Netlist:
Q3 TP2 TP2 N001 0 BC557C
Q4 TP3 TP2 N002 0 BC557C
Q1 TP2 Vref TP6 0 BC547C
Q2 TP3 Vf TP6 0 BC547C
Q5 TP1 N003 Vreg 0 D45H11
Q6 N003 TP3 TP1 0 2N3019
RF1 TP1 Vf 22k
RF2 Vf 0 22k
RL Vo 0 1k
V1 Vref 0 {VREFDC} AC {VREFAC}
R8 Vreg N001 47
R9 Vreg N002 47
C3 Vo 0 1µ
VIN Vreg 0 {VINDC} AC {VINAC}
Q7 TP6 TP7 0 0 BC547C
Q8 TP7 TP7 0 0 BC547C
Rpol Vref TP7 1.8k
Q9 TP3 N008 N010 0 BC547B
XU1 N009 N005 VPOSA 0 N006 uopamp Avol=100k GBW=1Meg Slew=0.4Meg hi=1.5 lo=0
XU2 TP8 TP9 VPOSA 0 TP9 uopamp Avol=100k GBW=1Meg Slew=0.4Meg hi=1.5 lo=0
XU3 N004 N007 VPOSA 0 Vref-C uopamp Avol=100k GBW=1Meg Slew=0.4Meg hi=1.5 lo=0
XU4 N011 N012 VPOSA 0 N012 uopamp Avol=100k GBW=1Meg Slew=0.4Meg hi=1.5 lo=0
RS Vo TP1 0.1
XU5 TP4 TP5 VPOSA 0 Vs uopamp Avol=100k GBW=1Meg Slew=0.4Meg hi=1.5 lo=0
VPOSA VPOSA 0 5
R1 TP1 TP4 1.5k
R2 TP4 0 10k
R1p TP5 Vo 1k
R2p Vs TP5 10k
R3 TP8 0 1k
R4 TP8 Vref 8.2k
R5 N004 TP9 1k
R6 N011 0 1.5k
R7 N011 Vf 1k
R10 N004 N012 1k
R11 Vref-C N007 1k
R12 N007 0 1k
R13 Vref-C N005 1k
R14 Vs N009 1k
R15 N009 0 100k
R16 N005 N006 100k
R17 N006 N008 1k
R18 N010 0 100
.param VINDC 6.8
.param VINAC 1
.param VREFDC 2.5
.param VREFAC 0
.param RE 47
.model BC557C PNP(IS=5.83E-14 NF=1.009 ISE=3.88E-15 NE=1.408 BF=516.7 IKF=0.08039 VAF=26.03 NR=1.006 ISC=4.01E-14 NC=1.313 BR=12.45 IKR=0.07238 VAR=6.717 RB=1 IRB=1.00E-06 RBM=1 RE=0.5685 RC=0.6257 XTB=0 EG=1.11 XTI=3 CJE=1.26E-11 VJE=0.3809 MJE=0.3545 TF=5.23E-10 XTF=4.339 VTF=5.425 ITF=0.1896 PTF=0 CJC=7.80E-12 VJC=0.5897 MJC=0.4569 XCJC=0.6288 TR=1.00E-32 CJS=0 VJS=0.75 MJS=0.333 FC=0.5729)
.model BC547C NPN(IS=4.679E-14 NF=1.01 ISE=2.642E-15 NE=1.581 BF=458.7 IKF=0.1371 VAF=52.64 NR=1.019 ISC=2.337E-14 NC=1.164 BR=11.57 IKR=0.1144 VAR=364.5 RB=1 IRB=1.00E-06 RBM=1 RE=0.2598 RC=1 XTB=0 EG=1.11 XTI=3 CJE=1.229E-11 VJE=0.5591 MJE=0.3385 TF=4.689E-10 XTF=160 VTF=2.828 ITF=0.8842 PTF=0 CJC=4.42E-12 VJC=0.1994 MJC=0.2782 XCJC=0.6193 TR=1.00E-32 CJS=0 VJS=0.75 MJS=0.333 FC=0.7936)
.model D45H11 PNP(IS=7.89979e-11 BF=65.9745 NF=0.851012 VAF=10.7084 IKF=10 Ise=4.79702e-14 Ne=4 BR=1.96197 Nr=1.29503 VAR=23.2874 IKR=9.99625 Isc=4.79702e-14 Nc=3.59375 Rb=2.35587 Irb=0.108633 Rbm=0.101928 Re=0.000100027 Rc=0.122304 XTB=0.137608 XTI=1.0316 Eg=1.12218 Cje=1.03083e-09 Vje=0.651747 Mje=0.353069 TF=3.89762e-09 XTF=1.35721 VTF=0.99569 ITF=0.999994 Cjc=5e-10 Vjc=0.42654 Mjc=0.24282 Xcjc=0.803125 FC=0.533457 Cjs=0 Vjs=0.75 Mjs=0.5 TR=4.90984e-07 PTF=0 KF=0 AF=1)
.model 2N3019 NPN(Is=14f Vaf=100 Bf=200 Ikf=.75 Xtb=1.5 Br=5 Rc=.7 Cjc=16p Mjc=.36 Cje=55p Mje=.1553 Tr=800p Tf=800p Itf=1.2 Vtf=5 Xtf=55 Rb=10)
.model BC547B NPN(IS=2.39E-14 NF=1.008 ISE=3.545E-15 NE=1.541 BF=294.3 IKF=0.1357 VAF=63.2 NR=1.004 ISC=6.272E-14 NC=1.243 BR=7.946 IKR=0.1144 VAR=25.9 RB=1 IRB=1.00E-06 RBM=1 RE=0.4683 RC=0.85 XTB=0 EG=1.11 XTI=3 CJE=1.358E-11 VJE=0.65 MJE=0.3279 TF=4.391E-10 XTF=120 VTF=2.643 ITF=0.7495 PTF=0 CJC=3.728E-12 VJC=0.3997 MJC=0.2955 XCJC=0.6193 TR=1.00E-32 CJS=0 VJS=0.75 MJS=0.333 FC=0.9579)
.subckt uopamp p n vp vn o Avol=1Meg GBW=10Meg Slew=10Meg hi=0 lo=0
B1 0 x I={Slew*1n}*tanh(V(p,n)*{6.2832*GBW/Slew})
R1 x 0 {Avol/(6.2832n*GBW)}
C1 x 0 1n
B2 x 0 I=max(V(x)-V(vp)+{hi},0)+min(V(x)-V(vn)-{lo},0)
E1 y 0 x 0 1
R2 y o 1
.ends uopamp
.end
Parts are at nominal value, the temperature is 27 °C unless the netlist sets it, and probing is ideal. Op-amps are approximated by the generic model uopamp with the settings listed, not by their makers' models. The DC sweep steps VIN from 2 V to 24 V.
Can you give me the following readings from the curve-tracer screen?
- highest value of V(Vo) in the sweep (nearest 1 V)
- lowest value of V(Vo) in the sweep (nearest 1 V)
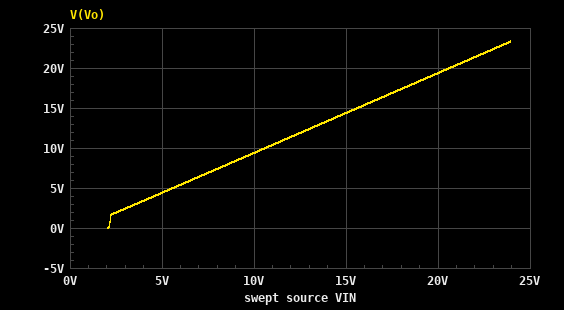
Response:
23 V
0 V
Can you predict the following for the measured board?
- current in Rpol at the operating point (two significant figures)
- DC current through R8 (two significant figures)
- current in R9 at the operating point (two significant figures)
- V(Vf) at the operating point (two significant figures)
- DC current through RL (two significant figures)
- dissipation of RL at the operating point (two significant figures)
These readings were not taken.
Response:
1.0 mA
840 µA
220 µA
570 mV
6.2 mA
38 mW
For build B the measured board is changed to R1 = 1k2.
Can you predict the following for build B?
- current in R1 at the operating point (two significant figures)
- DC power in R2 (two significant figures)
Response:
550 µA
3.1 mW
